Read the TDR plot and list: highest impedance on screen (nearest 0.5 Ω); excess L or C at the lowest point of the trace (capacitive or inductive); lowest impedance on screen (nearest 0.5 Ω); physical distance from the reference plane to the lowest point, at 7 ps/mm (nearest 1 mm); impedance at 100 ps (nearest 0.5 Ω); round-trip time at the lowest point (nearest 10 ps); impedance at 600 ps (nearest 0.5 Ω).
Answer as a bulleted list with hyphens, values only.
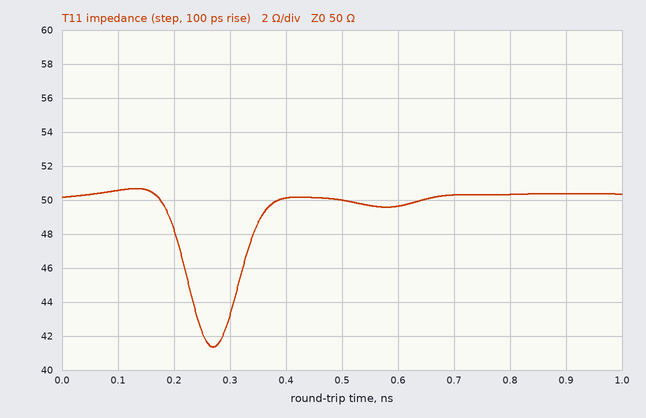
- 50.5 Ω
- capacitive
- 41.5 Ω
- 19 mm
- 50.5 Ω
- 270 ps
- 49.5 Ω
